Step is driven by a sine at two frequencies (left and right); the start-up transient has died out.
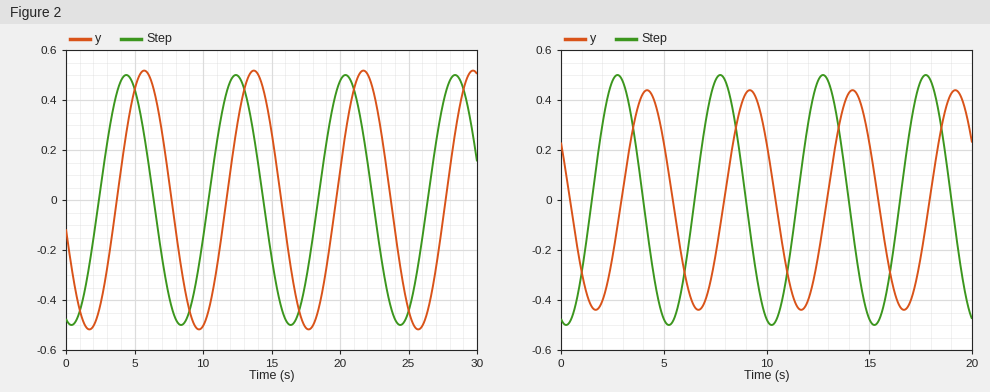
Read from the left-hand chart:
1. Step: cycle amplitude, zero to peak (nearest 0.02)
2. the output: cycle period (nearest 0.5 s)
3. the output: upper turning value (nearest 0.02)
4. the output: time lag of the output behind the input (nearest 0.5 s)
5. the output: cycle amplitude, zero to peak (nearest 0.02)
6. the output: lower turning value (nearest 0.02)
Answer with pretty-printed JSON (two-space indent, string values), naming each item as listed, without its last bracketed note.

{
  "Step: cycle amplitude, zero to peak": "0.50",
  "the output: cycle period": "8.0 s",
  "the output: upper turning value": "0.52",
  "the output: time lag of the output behind the input": "1.5 s",
  "the output: cycle amplitude, zero to peak": "0.52",
  "the output: lower turning value": "-0.52"
}
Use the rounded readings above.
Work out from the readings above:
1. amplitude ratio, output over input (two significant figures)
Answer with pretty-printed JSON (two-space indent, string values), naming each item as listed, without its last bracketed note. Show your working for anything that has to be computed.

{
  "amplitude ratio, output over input": "0.52 / 0.5 = 1.0"
}
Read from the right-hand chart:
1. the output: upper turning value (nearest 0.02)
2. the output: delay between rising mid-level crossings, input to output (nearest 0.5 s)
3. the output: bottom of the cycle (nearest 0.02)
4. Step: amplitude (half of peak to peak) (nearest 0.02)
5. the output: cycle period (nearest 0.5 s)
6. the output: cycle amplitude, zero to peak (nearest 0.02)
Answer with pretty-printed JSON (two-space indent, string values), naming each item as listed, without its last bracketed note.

{
  "the output: upper turning value": "0.44",
  "the output: delay between rising mid-level crossings, input to output": "1.5 s",
  "the output: bottom of the cycle": "-0.44",
  "Step: amplitude (half of peak to peak)": "0.50",
  "the output: cycle period": "5.0 s",
  "the output: cycle amplitude, zero to peak": "0.44"
}
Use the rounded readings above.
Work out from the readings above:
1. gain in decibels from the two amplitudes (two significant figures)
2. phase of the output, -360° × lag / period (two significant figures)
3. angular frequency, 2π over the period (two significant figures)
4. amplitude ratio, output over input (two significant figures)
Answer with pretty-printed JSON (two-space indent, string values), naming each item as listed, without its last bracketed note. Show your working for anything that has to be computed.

{
  "gain in decibels from the two amplitudes": "20 log10(0.44 / 0.5) = -1.1 dB",
  "phase of the output, -360° × lag / period": "-360 × 1.5 / 5 = -110°",
  "angular frequency, 2π over the period": "2π / 5 = 1.3 rad/s",
  "amplitude ratio, output over input": "0.44 / 0.5 = 0.88"
}
